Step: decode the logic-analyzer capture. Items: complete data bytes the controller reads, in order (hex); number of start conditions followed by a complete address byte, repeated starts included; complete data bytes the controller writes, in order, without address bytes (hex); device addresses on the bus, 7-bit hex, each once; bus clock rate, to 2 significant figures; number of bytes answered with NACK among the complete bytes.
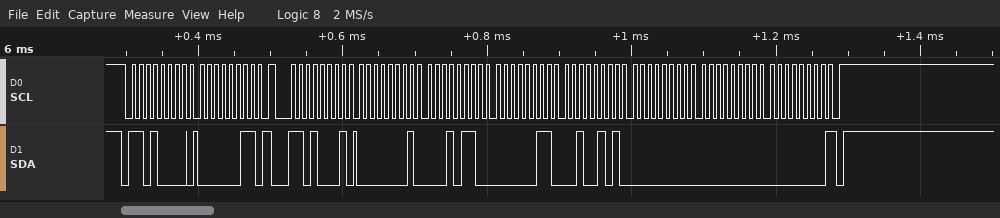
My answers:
01 16 03 25 00 00 00
2
03
0x68
100 kHz
1
